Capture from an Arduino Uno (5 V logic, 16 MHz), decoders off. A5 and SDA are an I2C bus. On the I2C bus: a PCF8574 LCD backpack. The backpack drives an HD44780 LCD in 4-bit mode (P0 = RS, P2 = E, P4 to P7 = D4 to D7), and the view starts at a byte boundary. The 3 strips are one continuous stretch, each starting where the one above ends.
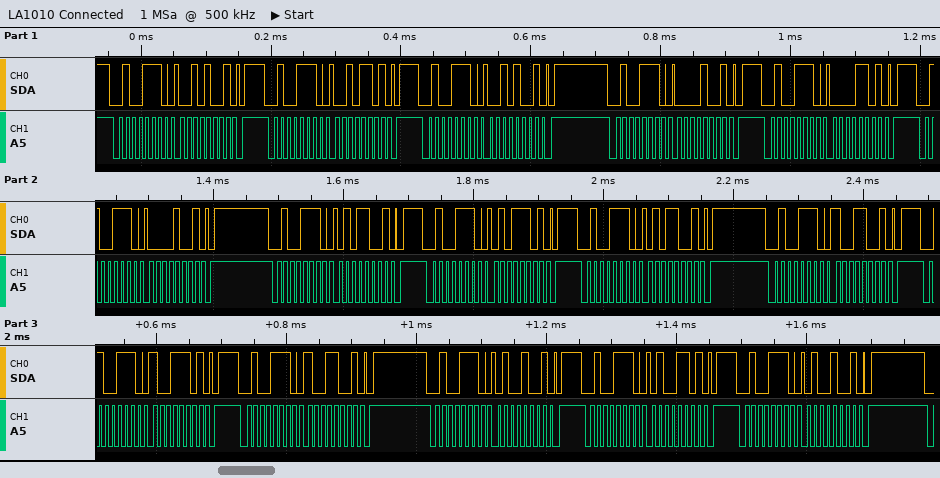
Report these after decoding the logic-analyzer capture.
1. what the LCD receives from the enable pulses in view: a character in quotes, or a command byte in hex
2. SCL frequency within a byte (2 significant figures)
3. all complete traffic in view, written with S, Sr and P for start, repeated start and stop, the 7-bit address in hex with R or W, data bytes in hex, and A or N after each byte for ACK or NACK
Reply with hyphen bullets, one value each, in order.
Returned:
- ' ' 'Y'
- 100 kHz
- S 27W A 29 A P S 27W A 2D A P S 27W A 29 A P S 27W A 09 A P S 27W A 0D A P S 27W A 09 A P S 27W A 59 A P S 27W A 5D A P S 27W A 59 A P S 27W A 99 A P S 27W A 9D A P S 27W A 99 A P S 27W A 49 A P S 27W A 4D A P S 27W A 49 A P
